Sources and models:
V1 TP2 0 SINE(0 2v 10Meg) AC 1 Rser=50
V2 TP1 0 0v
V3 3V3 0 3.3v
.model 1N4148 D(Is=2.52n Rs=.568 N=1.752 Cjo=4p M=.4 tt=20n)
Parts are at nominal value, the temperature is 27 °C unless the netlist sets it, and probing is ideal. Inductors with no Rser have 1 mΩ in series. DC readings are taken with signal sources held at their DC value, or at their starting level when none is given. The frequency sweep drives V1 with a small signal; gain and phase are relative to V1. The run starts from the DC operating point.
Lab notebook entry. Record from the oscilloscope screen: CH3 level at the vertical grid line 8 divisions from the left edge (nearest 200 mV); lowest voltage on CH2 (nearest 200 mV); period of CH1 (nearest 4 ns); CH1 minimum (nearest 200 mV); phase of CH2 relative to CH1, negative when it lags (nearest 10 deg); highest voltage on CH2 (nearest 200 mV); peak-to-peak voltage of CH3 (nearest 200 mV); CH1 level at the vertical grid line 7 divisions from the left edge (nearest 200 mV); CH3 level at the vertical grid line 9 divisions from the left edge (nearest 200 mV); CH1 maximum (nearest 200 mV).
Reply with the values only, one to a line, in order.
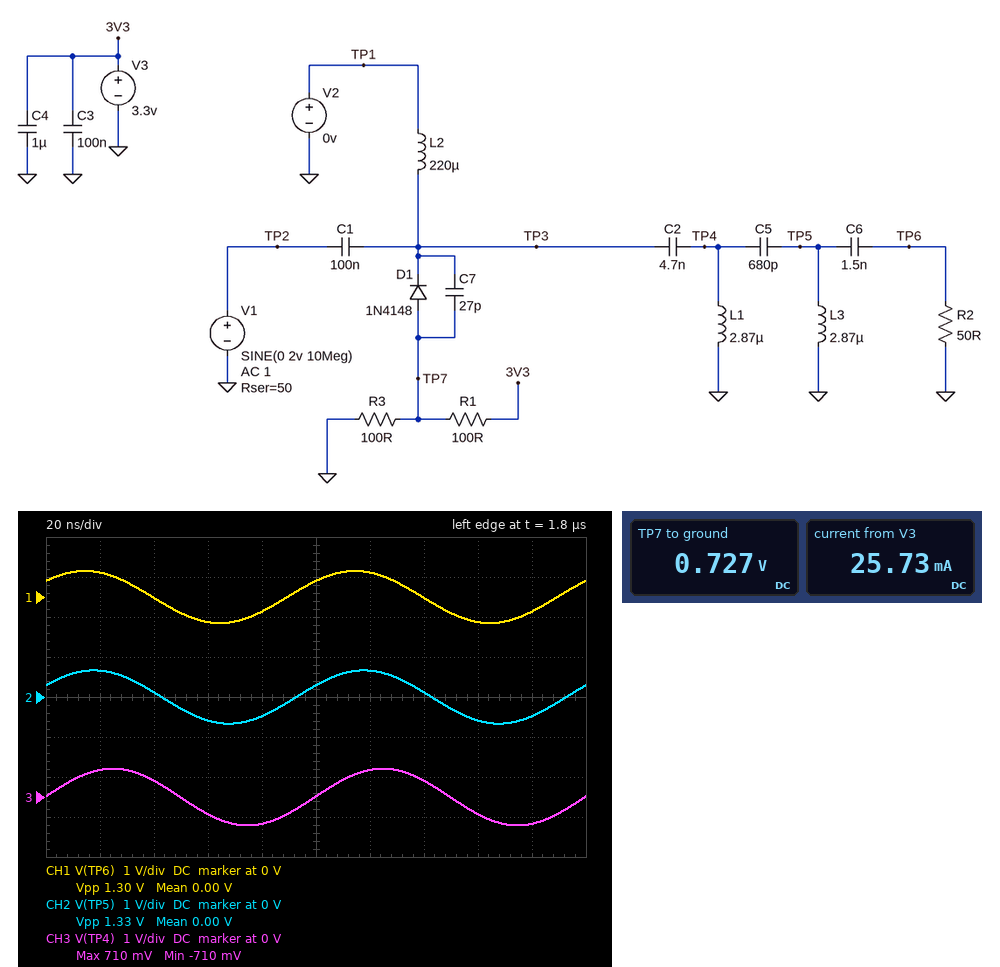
-400 mV
-600 mV
100 ns
-600 mV
-10 deg
600 mV
1.4 V
0 V
-600 mV
600 mV
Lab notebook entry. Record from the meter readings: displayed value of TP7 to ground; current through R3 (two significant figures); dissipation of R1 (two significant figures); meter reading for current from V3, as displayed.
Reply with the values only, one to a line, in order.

0.727 V
7.3 mA
66 mW
25.73 mA
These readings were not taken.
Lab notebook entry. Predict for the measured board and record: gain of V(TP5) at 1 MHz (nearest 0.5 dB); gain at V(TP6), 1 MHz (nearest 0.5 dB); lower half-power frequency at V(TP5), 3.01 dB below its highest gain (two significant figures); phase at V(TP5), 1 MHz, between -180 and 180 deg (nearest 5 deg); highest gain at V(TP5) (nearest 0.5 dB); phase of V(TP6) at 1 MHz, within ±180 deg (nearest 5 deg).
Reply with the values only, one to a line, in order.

-29.5 dB
-37.0 dB
1.8 MHz
-65 deg
-8.0 dB
0 deg
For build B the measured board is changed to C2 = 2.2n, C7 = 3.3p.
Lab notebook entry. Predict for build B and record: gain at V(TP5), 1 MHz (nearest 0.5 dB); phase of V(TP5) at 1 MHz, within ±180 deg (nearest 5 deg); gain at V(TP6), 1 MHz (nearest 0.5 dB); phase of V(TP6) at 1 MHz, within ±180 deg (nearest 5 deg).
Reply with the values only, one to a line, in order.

-35.5 dB
-30 deg
-43.0 dB
35 deg
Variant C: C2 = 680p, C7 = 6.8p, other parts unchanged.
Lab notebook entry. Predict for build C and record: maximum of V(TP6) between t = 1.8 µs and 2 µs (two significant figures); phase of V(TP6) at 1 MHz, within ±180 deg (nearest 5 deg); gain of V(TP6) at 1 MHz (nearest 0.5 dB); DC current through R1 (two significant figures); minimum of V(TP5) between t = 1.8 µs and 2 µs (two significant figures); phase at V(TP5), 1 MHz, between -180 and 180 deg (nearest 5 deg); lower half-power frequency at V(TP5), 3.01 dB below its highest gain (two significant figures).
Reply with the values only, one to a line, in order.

620 mV
55 deg
-54.0 dB
26 mA
-640 mV
-10 deg
2.0 MHz
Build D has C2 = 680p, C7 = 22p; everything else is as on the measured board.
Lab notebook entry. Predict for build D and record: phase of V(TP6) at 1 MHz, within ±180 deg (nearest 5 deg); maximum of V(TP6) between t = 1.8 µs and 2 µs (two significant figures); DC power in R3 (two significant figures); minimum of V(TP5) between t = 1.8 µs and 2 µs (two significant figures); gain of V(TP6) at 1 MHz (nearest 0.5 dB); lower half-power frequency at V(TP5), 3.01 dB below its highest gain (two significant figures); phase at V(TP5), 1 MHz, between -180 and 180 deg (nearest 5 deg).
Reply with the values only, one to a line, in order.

55 deg
620 mV
5.3 mW
-640 mV
-54.0 dB
2.0 MHz
-10 deg
